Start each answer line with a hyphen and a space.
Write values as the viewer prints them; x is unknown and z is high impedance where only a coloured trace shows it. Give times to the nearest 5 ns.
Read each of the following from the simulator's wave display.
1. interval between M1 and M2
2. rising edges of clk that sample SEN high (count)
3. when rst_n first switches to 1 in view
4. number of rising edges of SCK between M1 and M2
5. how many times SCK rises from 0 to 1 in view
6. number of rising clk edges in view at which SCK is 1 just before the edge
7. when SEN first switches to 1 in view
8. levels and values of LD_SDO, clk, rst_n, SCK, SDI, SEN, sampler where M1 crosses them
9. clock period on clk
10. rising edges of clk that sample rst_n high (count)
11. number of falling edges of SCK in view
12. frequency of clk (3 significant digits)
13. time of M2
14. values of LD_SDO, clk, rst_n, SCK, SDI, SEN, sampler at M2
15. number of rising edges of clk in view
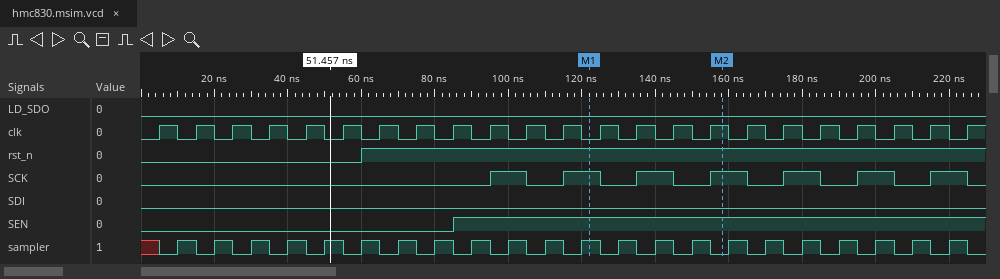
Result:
- 35 ns
- 14
- 60 ns
- 2
- 7
- 7
- 85 ns
- LD_SDO=0, clk=0, rst_n=1, SCK=1, SDI=0, SEN=1, sampler=1
- 10 ns
- 17
- 7
- 100 MHz
- 160 ns
- LD_SDO=0, clk=1, rst_n=1, SCK=1, SDI=0, SEN=1, sampler=0
- 23
